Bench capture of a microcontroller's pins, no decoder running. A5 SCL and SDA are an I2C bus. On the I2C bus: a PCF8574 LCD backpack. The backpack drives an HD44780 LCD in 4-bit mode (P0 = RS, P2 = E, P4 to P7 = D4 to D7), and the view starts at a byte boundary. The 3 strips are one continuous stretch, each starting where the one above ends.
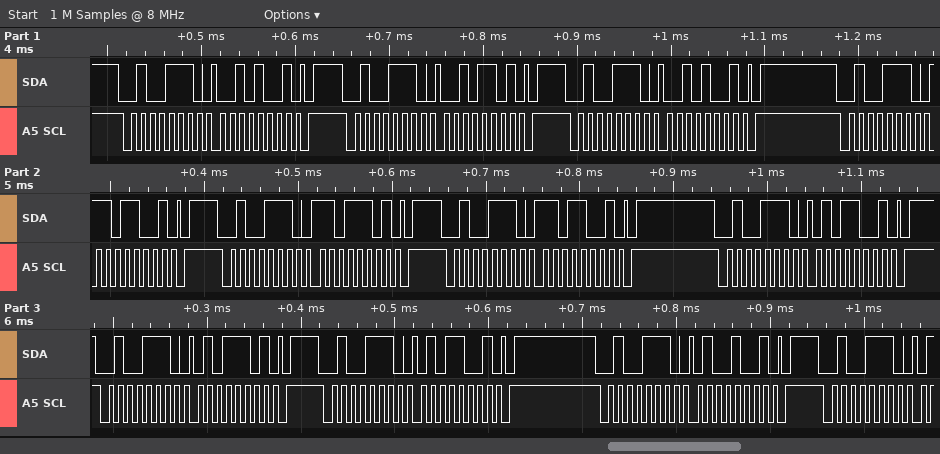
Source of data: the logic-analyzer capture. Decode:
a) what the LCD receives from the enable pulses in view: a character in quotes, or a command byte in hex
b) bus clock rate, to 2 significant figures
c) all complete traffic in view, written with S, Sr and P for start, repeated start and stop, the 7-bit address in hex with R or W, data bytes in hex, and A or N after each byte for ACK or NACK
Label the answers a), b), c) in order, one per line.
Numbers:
a) '-'
b) 100 kHz
c) S 27W A 29 A P S 27W A 2D A P S 27W A 29 A P S 27W A D9 A P S 27W A DD A P S 27W A D9 A P S 27W A 59 A P S 27W A 5D A P S 27W A 59 A P S 27W A 49 A P S 27W A
